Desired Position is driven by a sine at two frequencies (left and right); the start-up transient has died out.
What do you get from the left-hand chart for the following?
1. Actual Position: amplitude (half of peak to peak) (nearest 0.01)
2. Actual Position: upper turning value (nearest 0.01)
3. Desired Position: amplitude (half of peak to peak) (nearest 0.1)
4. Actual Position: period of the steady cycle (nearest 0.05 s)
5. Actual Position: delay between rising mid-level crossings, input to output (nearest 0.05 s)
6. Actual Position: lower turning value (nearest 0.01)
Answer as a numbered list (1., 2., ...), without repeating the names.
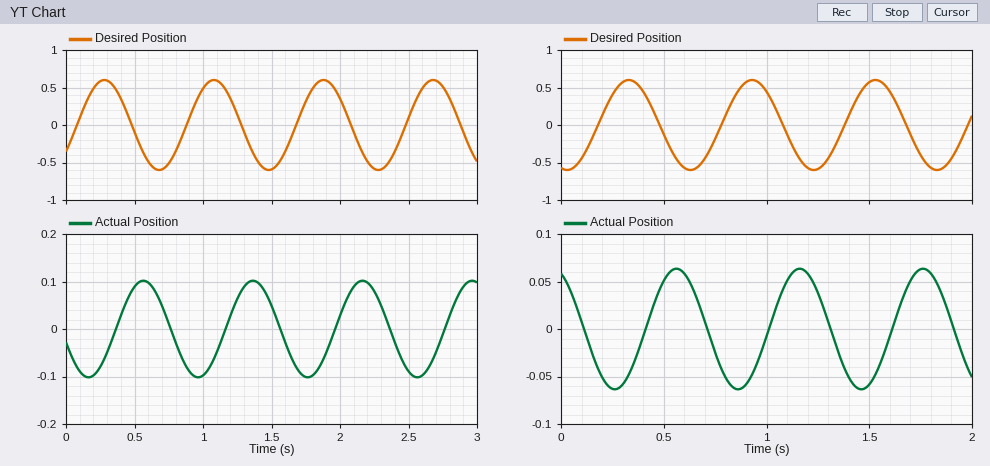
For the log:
1. 0.10
2. 0.10
3. 0.6
4. 0.80 s
5. 0.30 s
6. -0.10
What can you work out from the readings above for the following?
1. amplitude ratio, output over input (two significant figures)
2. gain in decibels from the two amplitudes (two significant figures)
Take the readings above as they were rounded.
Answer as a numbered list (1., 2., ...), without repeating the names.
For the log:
1. 0.17
2. -16 dB
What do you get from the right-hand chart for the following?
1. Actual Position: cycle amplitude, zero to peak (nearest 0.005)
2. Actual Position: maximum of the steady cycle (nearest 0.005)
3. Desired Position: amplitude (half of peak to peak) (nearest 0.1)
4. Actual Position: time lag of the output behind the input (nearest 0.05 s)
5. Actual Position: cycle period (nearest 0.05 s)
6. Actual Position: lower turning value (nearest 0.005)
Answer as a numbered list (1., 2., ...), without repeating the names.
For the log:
1. 0.065
2. 0.065
3. 0.6
4. 0.25 s
5. 0.60 s
6. -0.065
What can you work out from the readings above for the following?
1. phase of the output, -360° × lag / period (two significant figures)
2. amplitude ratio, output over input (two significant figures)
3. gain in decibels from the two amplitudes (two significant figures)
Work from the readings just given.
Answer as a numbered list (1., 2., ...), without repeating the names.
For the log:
1. -150°
2. 0.11
3. -19 dB
